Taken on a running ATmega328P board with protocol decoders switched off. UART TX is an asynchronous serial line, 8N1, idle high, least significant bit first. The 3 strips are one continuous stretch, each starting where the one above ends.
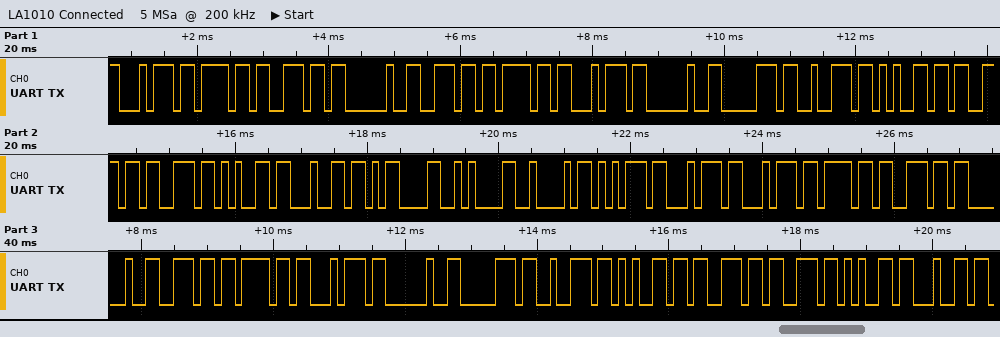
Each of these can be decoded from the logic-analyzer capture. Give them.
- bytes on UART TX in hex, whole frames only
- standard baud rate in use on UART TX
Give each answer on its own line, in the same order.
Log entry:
0x74 0x6F 0x6E 0x20 0x6E 0x6F 0x74 0x20 0x70 0x72 0x65 0x73 0x73 0x65 0x64 0x0D 0x0A 0x42 0x75 0x74 0x74 0x6F 0x6E 0x20 0x6E 0x6F 0x74 0x20 0x70 0x72 0x65 0x73 0x73 0x65 0x64
9600 baud
